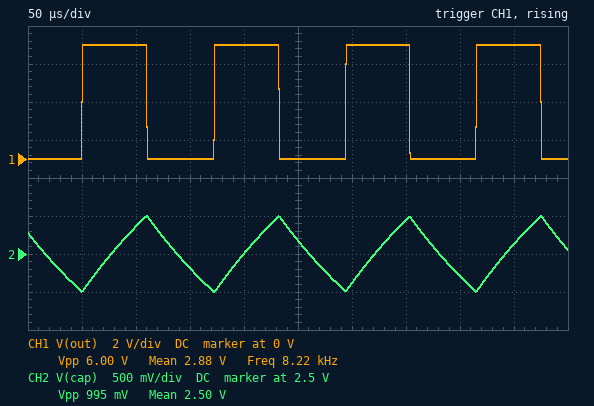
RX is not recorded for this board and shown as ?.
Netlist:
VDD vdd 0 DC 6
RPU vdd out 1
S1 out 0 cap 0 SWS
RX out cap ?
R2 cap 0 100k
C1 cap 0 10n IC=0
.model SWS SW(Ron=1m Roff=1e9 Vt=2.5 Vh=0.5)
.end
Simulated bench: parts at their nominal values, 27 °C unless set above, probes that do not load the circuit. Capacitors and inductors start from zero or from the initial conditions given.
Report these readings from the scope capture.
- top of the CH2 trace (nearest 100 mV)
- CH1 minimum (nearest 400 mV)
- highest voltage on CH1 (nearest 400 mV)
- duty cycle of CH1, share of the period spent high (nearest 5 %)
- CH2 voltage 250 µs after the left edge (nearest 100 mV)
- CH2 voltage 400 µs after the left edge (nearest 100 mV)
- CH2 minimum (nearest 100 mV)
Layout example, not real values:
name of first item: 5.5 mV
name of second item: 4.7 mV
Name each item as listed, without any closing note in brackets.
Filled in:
top of the CH2 trace: 3.0 V
CH1 minimum: 0 V
highest voltage on CH1: 6.0 V
duty cycle of CH1, share of the period spent high: 50 %
CH2 voltage 250 µs after the left edge: 2.7 V
CH2 voltage 400 µs after the left edge: 2.2 V
CH2 minimum: 2.0 V
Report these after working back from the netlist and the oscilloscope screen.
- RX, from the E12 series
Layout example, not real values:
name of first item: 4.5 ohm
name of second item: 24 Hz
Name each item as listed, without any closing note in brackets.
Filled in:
RX, from the E12 series: 18 kΩ
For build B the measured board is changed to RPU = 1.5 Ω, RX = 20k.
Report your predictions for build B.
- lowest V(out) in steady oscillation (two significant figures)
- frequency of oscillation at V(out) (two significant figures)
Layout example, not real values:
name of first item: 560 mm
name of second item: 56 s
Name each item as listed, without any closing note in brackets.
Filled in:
lowest V(out) in steady oscillation: 4.0 mV
frequency of oscillation at V(out): 7.4 kHz
